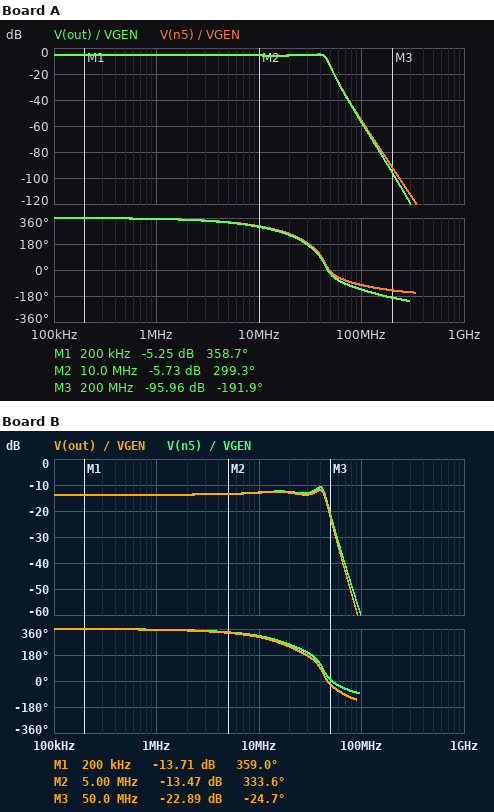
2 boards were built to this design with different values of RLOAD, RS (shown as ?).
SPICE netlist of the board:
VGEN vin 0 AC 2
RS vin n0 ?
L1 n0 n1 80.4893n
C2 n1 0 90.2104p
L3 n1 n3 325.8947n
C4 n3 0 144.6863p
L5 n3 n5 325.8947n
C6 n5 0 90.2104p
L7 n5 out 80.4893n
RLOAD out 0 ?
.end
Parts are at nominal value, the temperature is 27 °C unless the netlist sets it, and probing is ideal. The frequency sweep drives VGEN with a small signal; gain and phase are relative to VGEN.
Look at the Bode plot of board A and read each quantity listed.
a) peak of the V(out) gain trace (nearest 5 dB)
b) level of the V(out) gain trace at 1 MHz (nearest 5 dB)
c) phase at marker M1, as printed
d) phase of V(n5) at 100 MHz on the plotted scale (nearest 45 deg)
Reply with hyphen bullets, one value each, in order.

- -5 dB
- -5 dB
- 358.7 deg
- -90 deg
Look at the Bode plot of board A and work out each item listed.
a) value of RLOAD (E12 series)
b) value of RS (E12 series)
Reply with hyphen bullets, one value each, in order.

- 82 Ω
- 68 Ω
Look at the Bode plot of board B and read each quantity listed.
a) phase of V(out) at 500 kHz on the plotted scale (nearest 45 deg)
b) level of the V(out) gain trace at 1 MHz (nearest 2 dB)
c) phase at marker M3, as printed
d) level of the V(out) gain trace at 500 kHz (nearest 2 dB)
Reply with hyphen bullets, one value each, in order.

- 360 deg
- -14 dB
- -24.7 deg
- -14 dB
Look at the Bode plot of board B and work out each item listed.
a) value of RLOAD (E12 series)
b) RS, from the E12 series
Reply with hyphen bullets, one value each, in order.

- 39 Ω
- 150 Ω
